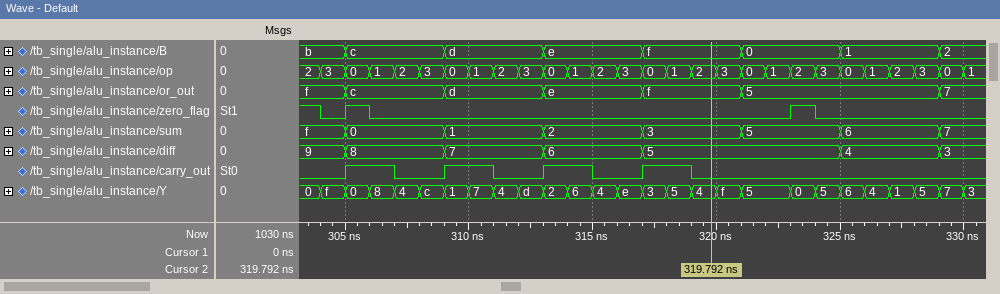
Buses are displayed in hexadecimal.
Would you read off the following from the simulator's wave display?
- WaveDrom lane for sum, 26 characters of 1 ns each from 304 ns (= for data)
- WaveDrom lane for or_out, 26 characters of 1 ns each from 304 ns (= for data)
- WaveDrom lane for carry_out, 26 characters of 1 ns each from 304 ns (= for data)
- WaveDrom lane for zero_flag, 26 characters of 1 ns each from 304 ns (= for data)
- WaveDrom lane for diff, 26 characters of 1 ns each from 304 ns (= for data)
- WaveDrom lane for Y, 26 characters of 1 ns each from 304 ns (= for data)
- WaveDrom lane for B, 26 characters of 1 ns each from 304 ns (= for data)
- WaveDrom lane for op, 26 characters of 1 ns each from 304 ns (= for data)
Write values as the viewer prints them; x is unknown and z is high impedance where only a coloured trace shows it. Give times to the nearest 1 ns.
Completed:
{name: 'sum', wave: '==...=...=...=...=...=...=', data: 'f 0 1 2 3 5 6 7'}
{name: 'or_out', wave: '==...=...=...=...=.......=', data: 'f c d e f 5 7'}
{name: 'carry_out', wave: '01.0.1.0.1.0.1.0..........'}
{name: 'zero_flag', wave: '010................10.....'}
{name: 'diff', wave: '==...=...=...=.......=...=', data: '9 8 7 6 5 4 3'}
{name: 'Y', wave: '==================.=======', data: 'f 0 8 4 c 1 7 4 d 2 6 4 e 3 5 4 f 5 0 5 6 4 1 5 7'}
{name: 'B', wave: '==...=...=...=...=...=...=', data: 'b c d e f 0 1 2'}
{name: 'op', wave: '==========================', data: '3 0 1 2 3 0 1 2 3 0 1 2 3 0 1 2 3 0 1 2 3 0 1 2 3 0'}
